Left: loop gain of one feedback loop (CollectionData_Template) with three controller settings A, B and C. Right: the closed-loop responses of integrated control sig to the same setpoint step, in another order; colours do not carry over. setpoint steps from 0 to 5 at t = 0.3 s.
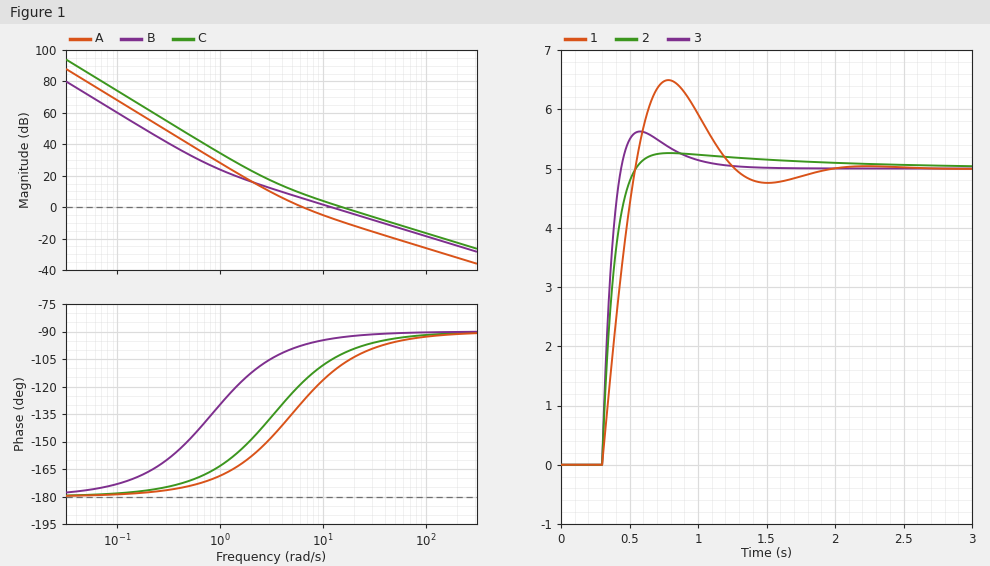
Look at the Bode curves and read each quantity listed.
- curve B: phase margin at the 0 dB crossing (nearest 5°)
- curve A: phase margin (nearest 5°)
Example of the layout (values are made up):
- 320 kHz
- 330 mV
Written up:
- 85°
- 50°
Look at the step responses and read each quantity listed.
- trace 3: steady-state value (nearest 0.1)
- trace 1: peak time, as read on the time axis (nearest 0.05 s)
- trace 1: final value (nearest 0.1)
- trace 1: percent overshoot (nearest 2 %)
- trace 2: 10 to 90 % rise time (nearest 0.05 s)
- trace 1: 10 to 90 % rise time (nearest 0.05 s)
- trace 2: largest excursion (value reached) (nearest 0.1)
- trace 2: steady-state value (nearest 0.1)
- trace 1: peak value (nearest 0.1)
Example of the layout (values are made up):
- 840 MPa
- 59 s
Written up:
- 5.0
- 0.80 s
- 5.0
- 30 %
- 0.15 s
- 0.20 s
- 5.3
- 5.0
- 6.5
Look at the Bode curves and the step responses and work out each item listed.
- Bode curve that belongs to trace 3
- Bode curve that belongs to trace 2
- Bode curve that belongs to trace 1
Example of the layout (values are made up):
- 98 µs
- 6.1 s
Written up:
- C
- B
- A
